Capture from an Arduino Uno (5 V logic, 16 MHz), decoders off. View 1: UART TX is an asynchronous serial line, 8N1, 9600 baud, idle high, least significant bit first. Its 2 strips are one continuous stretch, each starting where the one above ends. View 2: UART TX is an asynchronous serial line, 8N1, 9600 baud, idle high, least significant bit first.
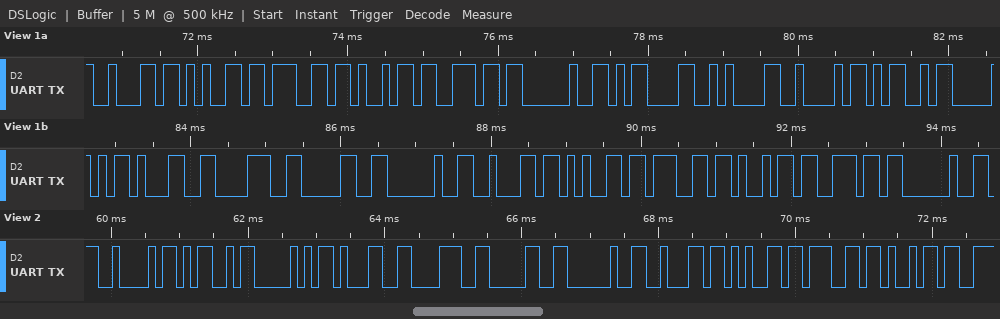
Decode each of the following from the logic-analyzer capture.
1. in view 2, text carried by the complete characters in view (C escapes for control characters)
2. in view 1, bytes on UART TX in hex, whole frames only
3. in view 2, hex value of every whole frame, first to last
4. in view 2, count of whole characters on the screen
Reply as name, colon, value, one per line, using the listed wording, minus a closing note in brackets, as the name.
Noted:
in view 2, text carried by the complete characters in view: "BMP180 begi"
in view 1, bytes on UART TX in hex, whole frames only: 62 65 67 69 6E 20 0D 0A 42 4D 50 31 38 30 20 62 65 67 69 6E 20
in view 2, hex value of every whole frame, first to last: 42 4D 50 31 38 30 20 62 65 67 69
in view 2, count of whole characters on the screen: 11
